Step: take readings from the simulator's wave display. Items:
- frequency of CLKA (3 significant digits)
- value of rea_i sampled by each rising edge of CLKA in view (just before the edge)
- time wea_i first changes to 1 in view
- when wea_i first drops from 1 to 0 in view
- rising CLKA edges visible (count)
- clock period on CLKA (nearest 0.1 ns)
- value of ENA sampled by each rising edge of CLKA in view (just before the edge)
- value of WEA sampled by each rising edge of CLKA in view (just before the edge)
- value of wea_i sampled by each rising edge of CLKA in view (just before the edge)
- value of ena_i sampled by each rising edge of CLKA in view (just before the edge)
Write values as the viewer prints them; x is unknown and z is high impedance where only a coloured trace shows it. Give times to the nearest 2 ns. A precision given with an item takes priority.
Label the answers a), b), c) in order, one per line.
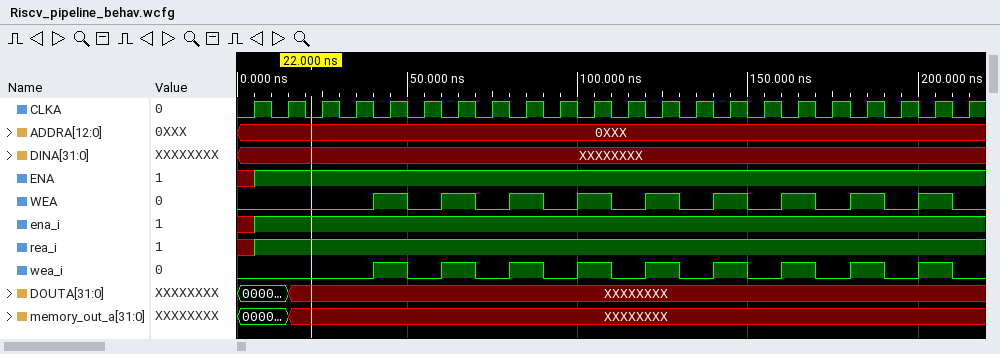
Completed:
a) 100 MHz
b) x 1 1 1 1 1 1 1 1 1 1 1 1 1 1 1 1 1 1 1 1 1
c) 40 ns
d) 50 ns
e) 22
f) 10 ns
g) x 1 1 1 1 1 1 1 1 1 1 1 1 1 1 1 1 1 1 1 1 1
h) 0 0 0 0 1 0 1 0 1 0 1 0 1 0 1 0 1 0 1 0 1 0
i) 0 0 0 0 1 0 1 0 1 0 1 0 1 0 1 0 1 0 1 0 1 0
j) x 1 1 1 1 1 1 1 1 1 1 1 1 1 1 1 1 1 1 1 1 1
